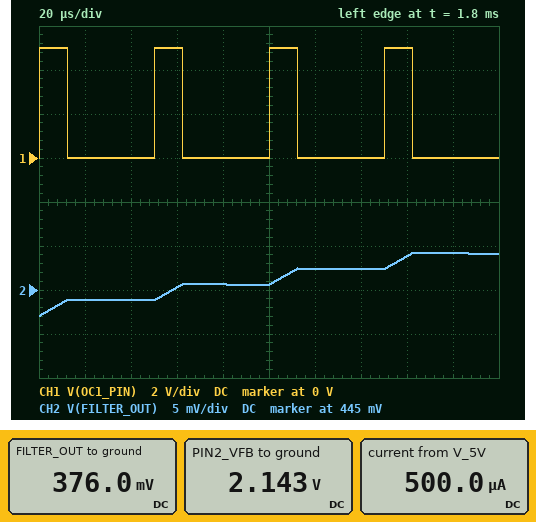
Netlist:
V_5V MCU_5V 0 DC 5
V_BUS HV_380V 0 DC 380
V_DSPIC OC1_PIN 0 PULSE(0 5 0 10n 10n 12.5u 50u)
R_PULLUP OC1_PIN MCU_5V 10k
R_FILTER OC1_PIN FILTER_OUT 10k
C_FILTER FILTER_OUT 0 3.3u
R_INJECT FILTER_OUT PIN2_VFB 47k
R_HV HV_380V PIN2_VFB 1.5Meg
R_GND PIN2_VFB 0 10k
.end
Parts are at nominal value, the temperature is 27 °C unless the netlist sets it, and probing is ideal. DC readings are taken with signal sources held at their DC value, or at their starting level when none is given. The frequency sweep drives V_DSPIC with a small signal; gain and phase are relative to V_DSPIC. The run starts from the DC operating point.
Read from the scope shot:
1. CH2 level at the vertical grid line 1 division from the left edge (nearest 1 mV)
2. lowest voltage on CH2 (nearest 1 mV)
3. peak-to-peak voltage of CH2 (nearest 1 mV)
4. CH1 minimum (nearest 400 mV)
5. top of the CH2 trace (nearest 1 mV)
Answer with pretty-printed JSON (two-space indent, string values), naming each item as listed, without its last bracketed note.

{
  "CH2 level at the vertical grid line 1 division from the left edge": "444 mV",
  "lowest voltage on CH2": "442 mV",
  "peak-to-peak voltage of CH2": "7 mV",
  "CH1 minimum": "0 V",
  "top of the CH2 trace": "449 mV"
}
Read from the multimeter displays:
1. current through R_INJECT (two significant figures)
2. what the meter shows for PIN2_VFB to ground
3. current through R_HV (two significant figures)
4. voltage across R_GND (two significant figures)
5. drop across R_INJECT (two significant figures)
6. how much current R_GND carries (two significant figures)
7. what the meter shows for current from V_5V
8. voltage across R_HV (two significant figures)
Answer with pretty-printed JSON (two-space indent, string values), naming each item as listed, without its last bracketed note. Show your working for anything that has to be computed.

{
  "current through R_INJECT": "(2.143 V - 376 mV) / 47 kΩ = 38 µA",
  "what the meter shows for PIN2_VFB to ground": "2.143 V",
  "current through R_HV": "(380 V - 2.143 V) / 1.5 MΩ = 250 µA",
  "voltage across R_GND": "2.143 V = 2.1 V",
  "drop across R_INJECT": "2.143 V - 376 mV = 1.8 V",
  "how much current R_GND carries": "(2.143 V) / 10 kΩ = 210 µA",
  "what the meter shows for current from V_5V": "500.0 µA",
  "voltage across R_HV": "380 V - 2.143 V = 380 V"
}
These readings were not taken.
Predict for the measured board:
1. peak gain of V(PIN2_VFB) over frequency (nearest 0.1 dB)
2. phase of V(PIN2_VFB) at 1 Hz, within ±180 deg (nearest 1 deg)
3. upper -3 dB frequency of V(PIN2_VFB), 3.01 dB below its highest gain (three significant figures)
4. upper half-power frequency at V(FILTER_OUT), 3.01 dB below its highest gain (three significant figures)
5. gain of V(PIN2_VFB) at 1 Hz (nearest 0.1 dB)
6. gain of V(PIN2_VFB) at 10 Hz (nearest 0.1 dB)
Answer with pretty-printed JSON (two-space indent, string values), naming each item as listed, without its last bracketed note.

{
  "peak gain of V(PIN2_VFB) over frequency": "-16.6 dB",
  "phase of V(PIN2_VFB) at 1 Hz, within ±180 deg": "-10 deg",
  "upper -3 dB frequency of V(PIN2_VFB), 3.01 dB below its highest gain": "5.67 Hz",
  "upper half-power frequency at V(FILTER_OUT), 3.01 dB below its highest gain": "5.67 Hz",
  "gain of V(PIN2_VFB) at 1 Hz": "-16.7 dB",
  "gain of V(PIN2_VFB) at 10 Hz": "-22.7 dB"
}
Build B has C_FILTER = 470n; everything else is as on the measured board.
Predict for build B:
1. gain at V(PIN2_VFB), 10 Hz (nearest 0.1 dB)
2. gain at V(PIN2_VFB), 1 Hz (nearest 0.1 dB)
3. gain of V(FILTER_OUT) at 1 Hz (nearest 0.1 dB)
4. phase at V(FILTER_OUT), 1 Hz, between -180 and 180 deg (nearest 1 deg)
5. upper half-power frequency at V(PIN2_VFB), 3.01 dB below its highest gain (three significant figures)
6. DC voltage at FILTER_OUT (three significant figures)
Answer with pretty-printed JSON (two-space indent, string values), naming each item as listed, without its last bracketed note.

{
  "gain at V(PIN2_VFB), 10 Hz": "-16.8 dB",
  "gain at V(PIN2_VFB), 1 Hz": "-16.6 dB",
  "gain of V(FILTER_OUT) at 1 Hz": "-1.4 dB",
  "phase at V(FILTER_OUT), 1 Hz, between -180 and 180 deg": "-1 deg",
  "upper half-power frequency at V(PIN2_VFB), 3.01 dB below its highest gain": "39.8 Hz",
  "DC voltage at FILTER_OUT": "376 mV"
}
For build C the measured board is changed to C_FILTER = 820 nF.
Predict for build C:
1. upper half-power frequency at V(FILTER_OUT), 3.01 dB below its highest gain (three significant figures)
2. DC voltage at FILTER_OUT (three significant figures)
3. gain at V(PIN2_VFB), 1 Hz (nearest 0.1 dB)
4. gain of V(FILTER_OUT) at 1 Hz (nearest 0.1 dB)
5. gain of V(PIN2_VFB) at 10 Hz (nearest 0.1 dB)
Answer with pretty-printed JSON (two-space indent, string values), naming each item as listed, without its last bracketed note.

{
  "upper half-power frequency at V(FILTER_OUT), 3.01 dB below its highest gain": "22.8 Hz",
  "DC voltage at FILTER_OUT": "376 mV",
  "gain at V(PIN2_VFB), 1 Hz": "-16.6 dB",
  "gain of V(FILTER_OUT) at 1 Hz": "-1.4 dB",
  "gain of V(PIN2_VFB) at 10 Hz": "-17.3 dB"
}
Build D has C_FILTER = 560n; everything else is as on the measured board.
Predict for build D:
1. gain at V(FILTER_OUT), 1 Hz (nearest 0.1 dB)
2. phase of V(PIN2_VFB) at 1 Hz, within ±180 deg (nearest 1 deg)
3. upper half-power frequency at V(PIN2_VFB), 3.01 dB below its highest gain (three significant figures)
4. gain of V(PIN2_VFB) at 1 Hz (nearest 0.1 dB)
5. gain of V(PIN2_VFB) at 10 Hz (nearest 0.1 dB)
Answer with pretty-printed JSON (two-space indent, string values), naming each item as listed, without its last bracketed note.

{
  "gain at V(FILTER_OUT), 1 Hz": "-1.4 dB",
  "phase of V(PIN2_VFB) at 1 Hz, within ±180 deg": "-2 deg",
  "upper half-power frequency at V(PIN2_VFB), 3.01 dB below its highest gain": "33.4 Hz",
  "gain of V(PIN2_VFB) at 1 Hz": "-16.6 dB",
  "gain of V(PIN2_VFB) at 10 Hz": "-16.9 dB"
}
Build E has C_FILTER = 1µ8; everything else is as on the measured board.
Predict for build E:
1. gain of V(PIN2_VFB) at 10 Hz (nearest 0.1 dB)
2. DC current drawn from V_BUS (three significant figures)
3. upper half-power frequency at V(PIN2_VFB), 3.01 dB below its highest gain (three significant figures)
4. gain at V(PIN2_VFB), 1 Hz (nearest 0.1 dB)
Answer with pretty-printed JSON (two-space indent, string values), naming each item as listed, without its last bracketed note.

{
  "gain of V(PIN2_VFB) at 10 Hz": "-19.4 dB",
  "DC current drawn from V_BUS": "252 µA",
  "upper half-power frequency at V(PIN2_VFB), 3.01 dB below its highest gain": "10.4 Hz",
  "gain at V(PIN2_VFB), 1 Hz": "-16.6 dB"
}
